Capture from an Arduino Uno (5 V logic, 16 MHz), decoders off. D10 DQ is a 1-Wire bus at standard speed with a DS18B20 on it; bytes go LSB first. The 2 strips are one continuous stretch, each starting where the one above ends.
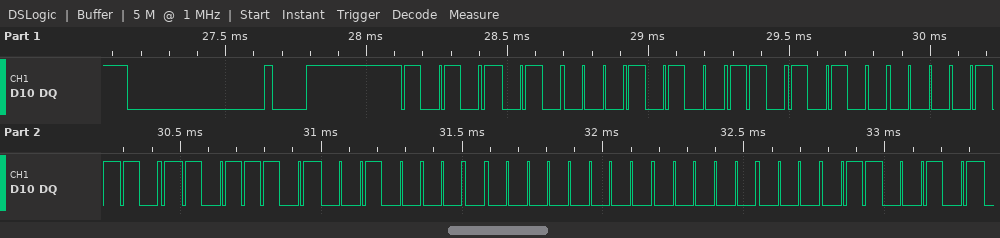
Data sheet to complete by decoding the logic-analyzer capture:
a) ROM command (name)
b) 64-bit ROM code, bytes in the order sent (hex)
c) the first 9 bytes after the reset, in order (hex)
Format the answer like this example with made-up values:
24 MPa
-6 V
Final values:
Match ROM
28 2B 70 BB 04 00 00 A6
55 28 2B 70 BB 04 00 00 A6
